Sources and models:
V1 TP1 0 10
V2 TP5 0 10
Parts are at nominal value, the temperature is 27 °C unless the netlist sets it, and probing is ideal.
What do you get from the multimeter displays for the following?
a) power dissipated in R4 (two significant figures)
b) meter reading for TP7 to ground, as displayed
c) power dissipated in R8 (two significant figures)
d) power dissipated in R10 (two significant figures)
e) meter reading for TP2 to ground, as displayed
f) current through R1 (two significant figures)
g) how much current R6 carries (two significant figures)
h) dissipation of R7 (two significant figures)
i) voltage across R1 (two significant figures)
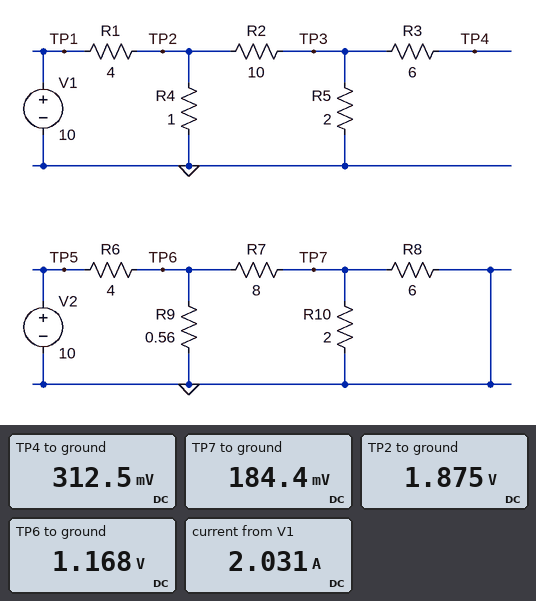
3.5 W
184.4 mV
5.7 mW
17 mW
1.875 V
2.0 A
2.2 A
120 mW
8.1 V
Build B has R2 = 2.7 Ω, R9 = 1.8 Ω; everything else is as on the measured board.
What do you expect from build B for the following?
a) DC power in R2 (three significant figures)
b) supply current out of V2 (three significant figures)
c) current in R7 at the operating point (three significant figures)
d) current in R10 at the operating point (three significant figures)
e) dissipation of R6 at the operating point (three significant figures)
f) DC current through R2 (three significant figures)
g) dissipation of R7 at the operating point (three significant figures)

357 mW
1.81 A
289 mA
217 mA
13.2 W
364 mA
668 mW
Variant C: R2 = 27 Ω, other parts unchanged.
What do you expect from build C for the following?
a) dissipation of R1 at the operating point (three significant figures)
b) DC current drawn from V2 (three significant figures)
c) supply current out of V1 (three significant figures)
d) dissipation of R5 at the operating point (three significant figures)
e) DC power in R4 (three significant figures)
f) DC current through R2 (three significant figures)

16.2 W
2.21 A
2.01 A
9.01 mW
3.79 W
67.1 mA
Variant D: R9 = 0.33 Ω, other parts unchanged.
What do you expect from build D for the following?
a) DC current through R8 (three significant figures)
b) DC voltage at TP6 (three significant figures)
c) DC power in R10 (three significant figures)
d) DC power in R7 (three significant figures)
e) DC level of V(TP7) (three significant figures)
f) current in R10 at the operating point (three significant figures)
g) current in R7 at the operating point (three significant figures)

19.4 mA
738 mV
6.80 mW
48.3 mW
117 mV
58.3 mA
77.7 mA
